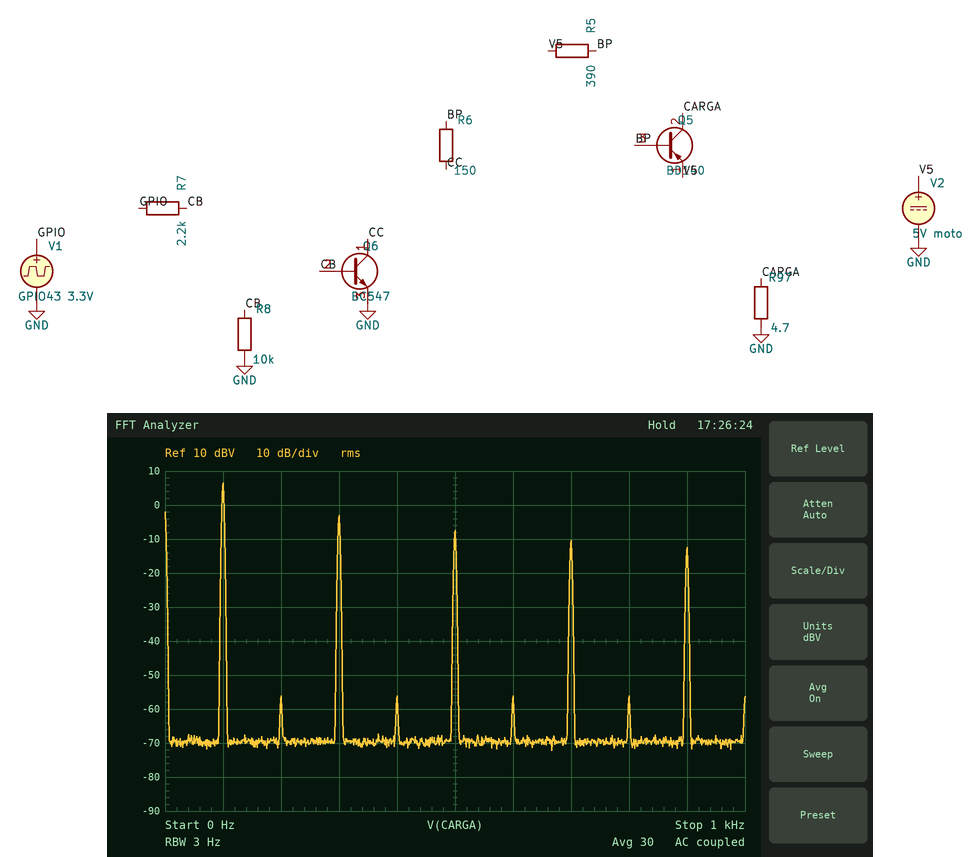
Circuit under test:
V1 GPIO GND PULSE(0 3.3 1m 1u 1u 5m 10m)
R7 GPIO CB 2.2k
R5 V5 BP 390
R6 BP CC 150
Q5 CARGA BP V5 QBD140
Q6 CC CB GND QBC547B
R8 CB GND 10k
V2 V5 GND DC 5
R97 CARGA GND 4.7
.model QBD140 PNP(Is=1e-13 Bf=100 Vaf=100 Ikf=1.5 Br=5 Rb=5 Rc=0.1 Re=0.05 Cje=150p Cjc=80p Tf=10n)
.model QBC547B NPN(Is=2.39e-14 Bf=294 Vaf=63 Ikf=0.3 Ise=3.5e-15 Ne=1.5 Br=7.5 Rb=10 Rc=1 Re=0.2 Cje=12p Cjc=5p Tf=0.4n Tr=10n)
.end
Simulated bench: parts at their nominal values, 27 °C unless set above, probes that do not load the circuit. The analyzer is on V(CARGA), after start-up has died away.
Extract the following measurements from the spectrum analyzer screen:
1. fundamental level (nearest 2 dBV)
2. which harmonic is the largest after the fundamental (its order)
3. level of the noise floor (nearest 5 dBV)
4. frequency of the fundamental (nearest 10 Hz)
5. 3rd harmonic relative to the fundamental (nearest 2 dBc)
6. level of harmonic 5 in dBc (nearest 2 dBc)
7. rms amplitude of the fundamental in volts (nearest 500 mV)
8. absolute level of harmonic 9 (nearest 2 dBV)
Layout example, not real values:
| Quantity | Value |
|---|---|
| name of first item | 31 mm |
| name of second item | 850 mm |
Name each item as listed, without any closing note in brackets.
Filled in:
| Quantity | Value |
|---|---|
| fundamental level | 6 dBV |
| which harmonic is the largest after the fundamental | 3 |
| level of the noise floor | -70 dBV |
| frequency of the fundamental | 100 Hz |
| 3rd harmonic relative to the fundamental | -10 dBc |
| level of harmonic 5 in dBc | -14 dBc |
| rms amplitude of the fundamental in volts | 2.0 V |
| absolute level of harmonic 9 | -12 dBV |
